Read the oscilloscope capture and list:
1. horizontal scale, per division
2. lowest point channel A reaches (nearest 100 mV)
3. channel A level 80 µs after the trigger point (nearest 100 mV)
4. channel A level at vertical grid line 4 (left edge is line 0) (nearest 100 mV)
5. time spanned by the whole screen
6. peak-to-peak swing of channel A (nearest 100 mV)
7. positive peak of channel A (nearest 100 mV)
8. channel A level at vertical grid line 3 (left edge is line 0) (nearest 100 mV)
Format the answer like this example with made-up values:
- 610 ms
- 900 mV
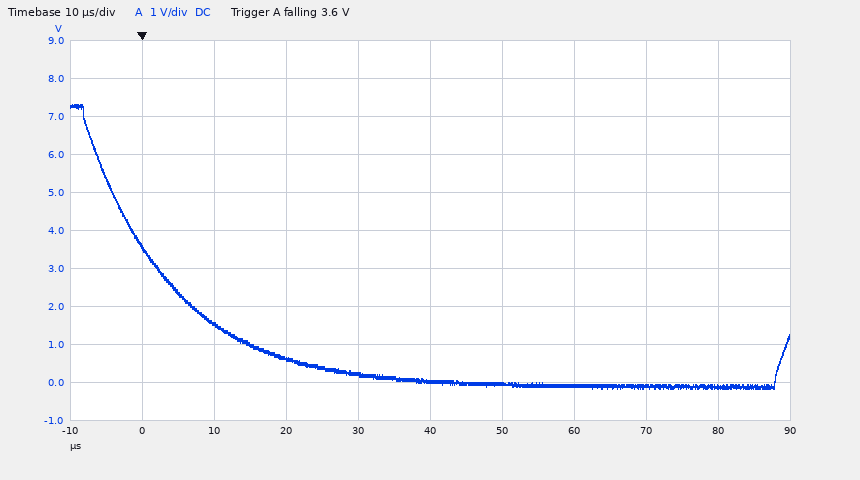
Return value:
- 10 µs
- -200 mV
- -100 mV
- 200 mV
- 100 µs
- 7.5 V
- 7.3 V
- 600 mV
